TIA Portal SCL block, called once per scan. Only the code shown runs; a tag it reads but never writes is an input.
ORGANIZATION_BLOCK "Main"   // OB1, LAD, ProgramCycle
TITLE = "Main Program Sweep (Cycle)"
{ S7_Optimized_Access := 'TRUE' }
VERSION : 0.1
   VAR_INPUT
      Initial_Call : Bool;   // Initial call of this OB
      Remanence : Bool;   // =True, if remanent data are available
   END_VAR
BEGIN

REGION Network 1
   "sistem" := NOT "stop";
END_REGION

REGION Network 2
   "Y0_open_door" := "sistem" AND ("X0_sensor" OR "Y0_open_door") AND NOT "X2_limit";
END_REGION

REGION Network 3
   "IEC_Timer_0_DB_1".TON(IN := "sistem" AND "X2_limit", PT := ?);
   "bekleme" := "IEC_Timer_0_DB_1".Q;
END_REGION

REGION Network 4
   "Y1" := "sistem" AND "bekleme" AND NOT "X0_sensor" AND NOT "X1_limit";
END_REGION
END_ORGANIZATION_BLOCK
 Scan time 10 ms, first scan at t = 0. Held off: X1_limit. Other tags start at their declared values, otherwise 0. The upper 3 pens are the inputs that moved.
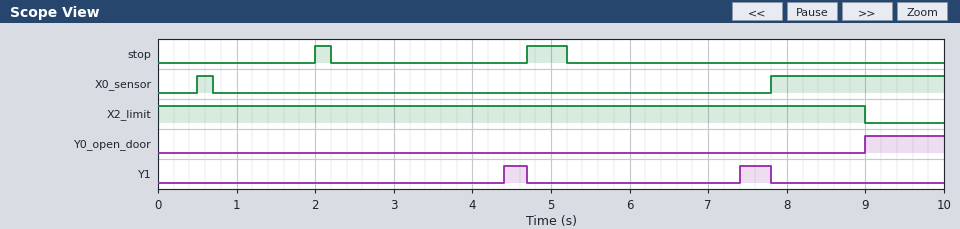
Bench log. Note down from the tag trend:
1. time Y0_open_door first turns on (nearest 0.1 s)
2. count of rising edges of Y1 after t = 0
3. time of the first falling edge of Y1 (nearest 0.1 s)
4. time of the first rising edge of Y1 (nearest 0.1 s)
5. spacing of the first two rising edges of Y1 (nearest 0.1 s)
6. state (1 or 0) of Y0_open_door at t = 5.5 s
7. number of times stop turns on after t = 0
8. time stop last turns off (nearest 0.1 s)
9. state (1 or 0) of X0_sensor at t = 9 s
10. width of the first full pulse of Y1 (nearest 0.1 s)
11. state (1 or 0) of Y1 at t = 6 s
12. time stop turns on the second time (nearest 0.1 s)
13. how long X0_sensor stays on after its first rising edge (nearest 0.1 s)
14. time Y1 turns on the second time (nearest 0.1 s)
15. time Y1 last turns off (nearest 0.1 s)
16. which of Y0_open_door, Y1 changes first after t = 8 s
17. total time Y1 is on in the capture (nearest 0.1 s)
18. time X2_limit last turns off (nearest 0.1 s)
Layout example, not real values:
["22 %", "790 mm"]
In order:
["9.0 s", "2", "4.7 s", "4.4 s", "3.0 s", "0", "2", "5.2 s", "1", "0.3 s", "0", "4.7 s", "0.2 s", "7.4 s", "7.8 s", "Y0_open_door", "0.7 s", "9.0 s"]
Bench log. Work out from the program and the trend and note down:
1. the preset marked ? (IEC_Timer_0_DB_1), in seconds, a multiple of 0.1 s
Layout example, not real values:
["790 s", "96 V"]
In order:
["2.2 s"]
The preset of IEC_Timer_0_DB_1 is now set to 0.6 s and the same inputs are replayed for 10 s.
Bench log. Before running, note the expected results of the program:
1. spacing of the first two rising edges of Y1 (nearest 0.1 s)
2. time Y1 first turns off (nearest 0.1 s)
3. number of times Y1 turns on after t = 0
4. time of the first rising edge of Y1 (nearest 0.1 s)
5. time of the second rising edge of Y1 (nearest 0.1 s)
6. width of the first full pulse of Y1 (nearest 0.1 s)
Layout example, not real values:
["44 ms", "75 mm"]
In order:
["2.1 s", "2.0 s", "3", "0.7 s", "2.8 s", "1.3 s"]
